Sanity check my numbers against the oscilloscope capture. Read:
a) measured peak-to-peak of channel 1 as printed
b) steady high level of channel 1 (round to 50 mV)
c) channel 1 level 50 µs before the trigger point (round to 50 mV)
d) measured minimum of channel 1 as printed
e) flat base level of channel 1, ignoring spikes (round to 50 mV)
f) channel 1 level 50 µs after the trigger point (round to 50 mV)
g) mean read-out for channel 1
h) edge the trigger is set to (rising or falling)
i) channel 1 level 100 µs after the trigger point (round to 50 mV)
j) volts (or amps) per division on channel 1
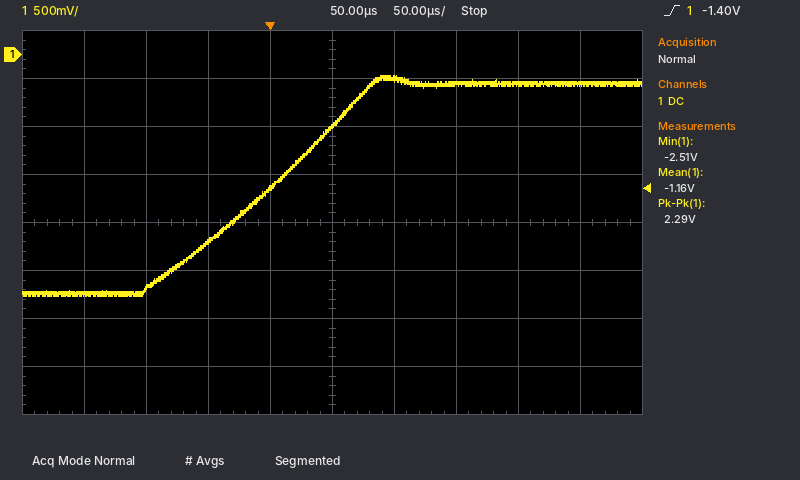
2.29 V
-300 mV
-1.95 V
-2.51 V
-2.50 V
-750 mV
-1.16 V
rising
-250 mV
500 mV
